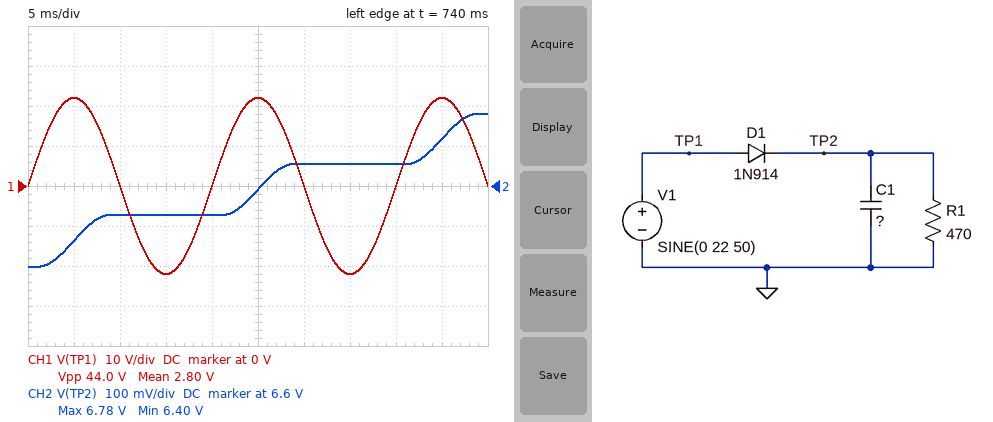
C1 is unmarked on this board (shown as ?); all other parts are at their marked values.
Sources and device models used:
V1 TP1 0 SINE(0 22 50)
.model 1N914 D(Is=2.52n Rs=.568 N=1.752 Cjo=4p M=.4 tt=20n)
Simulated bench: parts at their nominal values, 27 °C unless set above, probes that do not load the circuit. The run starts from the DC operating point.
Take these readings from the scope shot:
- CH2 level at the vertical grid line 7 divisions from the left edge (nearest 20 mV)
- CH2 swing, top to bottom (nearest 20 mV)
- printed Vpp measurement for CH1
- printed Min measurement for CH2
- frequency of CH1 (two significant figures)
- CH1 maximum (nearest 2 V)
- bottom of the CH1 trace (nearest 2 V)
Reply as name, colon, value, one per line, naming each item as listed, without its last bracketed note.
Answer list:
CH2 level at the vertical grid line 7 divisions from the left edge: 6.66 V
CH2 swing, top to bottom: 380 mV
printed Vpp measurement for CH1: 44.0 V
printed Min measurement for CH2: 6.40 V
frequency of CH1: 50 Hz
CH1 maximum: 22 V
bottom of the CH1 trace: -22 V
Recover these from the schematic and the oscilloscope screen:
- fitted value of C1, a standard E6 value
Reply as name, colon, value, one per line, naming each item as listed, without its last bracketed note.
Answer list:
fitted value of C1, a standard E6 value: 1 F
